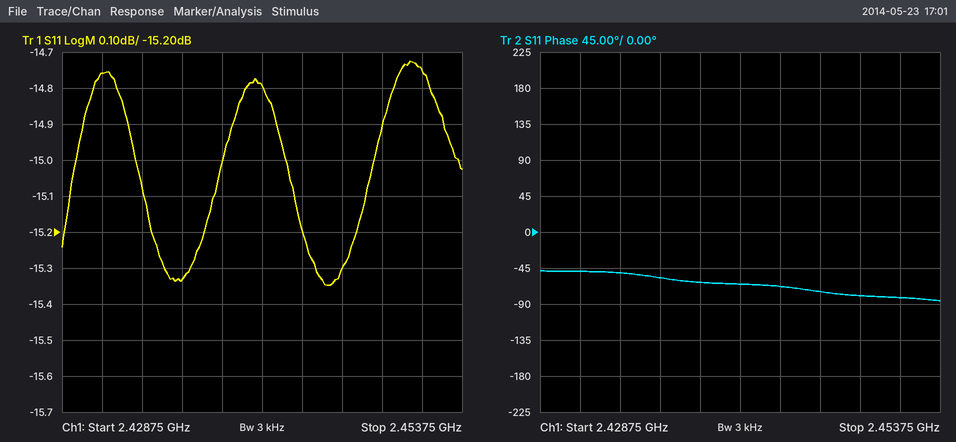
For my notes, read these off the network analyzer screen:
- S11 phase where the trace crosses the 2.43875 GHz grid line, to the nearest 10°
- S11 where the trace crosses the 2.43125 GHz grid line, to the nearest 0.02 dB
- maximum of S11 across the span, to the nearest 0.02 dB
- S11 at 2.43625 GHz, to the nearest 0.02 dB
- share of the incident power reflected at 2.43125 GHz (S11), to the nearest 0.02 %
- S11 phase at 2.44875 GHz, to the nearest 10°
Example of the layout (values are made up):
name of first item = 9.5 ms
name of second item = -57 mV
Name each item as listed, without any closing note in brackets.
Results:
S11 phase where the trace crosses the 2.43875 GHz grid line, to the nearest 10° = -60°
S11 where the trace crosses the 2.43125 GHz grid line, to the nearest 0.02 dB = -14.76 dB
maximum of S11 across the span, to the nearest 0.02 dB = -14.72 dB
S11 at 2.43625 GHz, to the nearest 0.02 dB = -15.34 dB
share of the incident power reflected at 2.43125 GHz (S11), to the nearest 0.02 % = 3.34 %
S11 phase at 2.44875 GHz, to the nearest 10° = -80°
